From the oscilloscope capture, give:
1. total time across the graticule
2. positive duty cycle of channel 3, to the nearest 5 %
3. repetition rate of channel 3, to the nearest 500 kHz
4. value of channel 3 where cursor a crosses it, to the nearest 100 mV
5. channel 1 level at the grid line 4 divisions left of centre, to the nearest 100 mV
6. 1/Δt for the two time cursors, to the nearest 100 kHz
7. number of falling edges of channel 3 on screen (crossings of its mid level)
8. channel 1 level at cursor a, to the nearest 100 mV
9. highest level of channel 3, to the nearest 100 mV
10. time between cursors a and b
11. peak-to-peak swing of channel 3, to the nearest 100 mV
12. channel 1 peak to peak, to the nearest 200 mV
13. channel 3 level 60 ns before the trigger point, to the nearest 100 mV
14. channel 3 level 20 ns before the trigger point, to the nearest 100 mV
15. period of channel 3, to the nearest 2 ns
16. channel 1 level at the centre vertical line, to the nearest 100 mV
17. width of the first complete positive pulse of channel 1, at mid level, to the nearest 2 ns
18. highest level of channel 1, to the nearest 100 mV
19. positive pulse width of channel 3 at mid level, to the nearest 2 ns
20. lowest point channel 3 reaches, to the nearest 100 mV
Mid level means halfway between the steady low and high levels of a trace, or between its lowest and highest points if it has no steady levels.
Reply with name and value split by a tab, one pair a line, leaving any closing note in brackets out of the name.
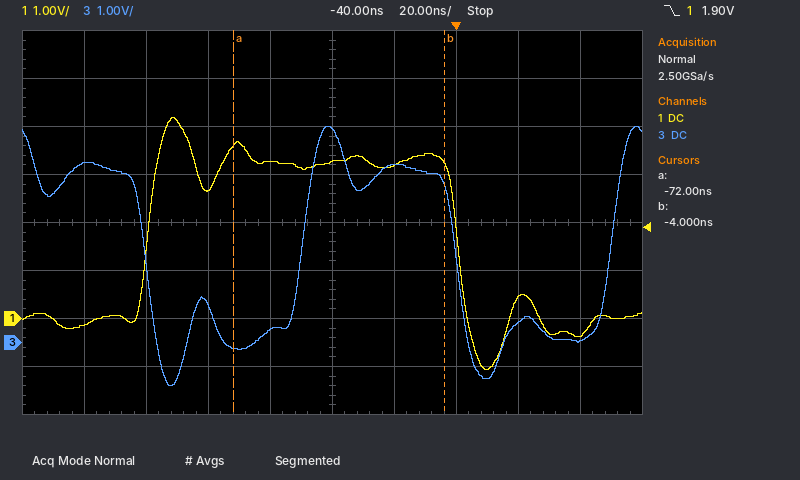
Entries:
total time across the graticule	200 ns
positive duty cycle of channel 3, to the nearest 5 %	50 %
repetition rate of channel 3, to the nearest 500 kHz	10.0 MHz
value of channel 3 where cursor a crosses it, to the nearest 100 mV	-100 mV
channel 1 level at the grid line 4 divisions left of centre, to the nearest 100 mV	-100 mV
1/Δt for the two time cursors, to the nearest 100 kHz	14.7 MHz
number of falling edges of channel 3 on screen	2
channel 1 level at cursor a, to the nearest 100 mV	3.6 V
highest level of channel 3, to the nearest 100 mV	4.5 V
time between cursors a and b	68 ns
peak-to-peak swing of channel 3, to the nearest 100 mV	5.4 V
channel 1 peak to peak, to the nearest 200 mV	5.2 V
channel 3 level 60 ns before the trigger point, to the nearest 100 mV	300 mV
channel 3 level 20 ns before the trigger point, to the nearest 100 mV	3.7 V
period of channel 3, to the nearest 2 ns	100 ns
channel 1 level at the centre vertical line, to the nearest 100 mV	3.3 V
width of the first complete positive pulse of channel 1, at mid level, to the nearest 2 ns	100 ns
highest level of channel 1, to the nearest 100 mV	4.2 V
positive pulse width of channel 3 at mid level, to the nearest 2 ns	50 ns
lowest point channel 3 reaches, to the nearest 100 mV	-900 mV
